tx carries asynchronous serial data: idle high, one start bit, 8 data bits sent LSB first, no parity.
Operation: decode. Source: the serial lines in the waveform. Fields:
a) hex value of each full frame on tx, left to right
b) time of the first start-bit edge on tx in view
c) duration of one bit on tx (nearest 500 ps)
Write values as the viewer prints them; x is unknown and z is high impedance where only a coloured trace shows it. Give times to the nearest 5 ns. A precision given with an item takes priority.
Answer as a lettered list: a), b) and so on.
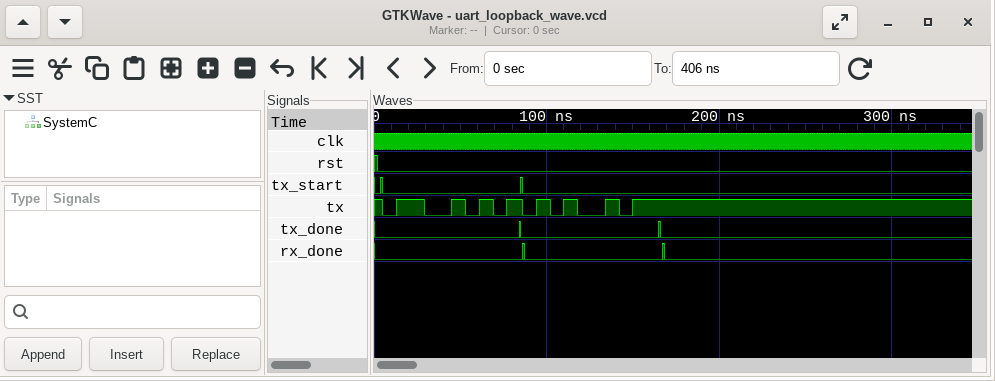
a) 53, A5
b) 5 ns
c) 8000 ps
